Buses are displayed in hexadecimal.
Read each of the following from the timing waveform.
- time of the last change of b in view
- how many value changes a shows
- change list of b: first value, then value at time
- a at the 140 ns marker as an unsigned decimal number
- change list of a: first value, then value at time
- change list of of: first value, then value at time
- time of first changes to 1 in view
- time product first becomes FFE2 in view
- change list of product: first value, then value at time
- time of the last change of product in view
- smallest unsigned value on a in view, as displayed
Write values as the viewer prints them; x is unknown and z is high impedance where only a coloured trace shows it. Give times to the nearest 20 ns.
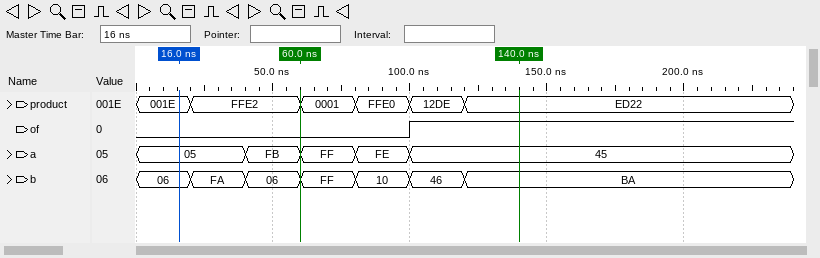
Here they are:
120 ns
4
06, FA at 20 ns, 06 at 40 ns, FF at 60 ns, 10 at 80 ns, 46 at 100 ns, BA at 120 ns
69
05, FB at 40 ns, FF at 60 ns, FE at 80 ns, 45 at 100 ns
0, 1 at 100 ns
100 ns
20 ns
001E, FFE2 at 20 ns, 0001 at 60 ns, FFE0 at 80 ns, 12DE at 100 ns, ED22 at 120 ns
120 ns
05
